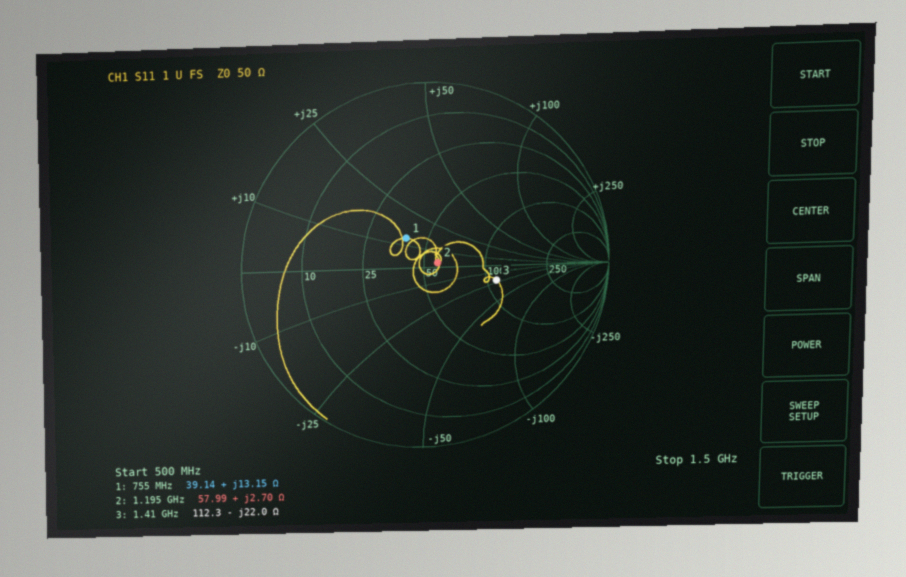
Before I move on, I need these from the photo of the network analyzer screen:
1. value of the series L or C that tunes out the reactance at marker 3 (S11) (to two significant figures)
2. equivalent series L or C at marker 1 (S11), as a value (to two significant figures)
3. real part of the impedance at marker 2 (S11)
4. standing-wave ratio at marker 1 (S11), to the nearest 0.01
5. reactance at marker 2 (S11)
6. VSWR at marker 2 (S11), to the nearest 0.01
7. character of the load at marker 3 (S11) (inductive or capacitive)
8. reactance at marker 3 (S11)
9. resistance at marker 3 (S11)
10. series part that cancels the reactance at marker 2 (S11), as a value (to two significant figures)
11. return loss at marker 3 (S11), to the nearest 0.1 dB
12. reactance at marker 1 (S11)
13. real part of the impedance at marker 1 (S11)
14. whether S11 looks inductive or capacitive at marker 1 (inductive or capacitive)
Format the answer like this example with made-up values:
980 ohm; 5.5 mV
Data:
2.5 nH; 2.8 nH; 57.99 Ω; 1.47; +2.70 Ω; 1.17; capacitive; -22.0 Ω; 112.3 Ω; 49 pF; 7.9 dB; +13.15 Ω; 39.14 Ω; inductive
